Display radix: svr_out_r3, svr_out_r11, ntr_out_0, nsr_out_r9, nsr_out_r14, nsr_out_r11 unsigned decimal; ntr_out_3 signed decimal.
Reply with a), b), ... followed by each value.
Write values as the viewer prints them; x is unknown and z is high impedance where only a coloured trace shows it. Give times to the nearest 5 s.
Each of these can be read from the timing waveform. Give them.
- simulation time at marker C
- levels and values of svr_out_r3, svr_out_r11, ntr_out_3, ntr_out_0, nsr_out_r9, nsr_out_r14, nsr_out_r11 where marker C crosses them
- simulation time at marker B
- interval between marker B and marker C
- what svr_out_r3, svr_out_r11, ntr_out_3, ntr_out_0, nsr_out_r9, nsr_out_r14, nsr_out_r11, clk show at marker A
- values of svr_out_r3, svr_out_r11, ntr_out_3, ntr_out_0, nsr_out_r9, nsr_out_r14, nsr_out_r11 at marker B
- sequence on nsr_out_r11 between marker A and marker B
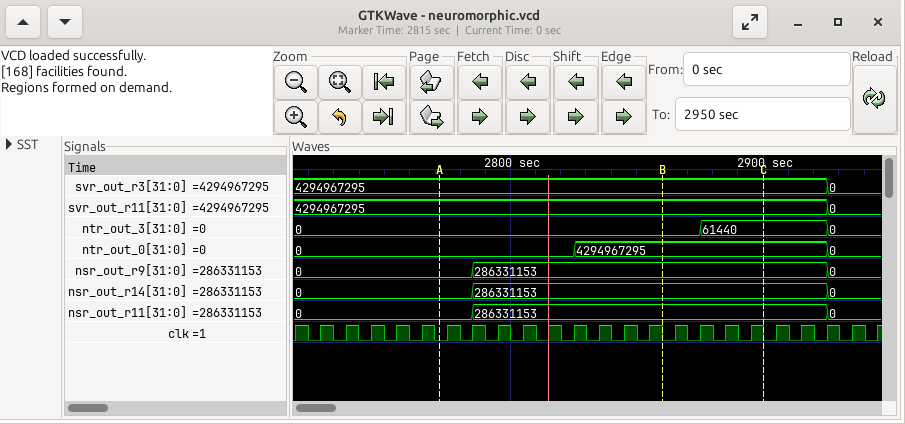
a) 2900 s
b) svr_out_r3=4294967295, svr_out_r11=4294967295, ntr_out_3=61440, ntr_out_0=4294967295, nsr_out_r9=286331153, nsr_out_r14=286331153, nsr_out_r11=286331153
c) 2860 s
d) 40 s
e) svr_out_r3=4294967295, svr_out_r11=4294967295, ntr_out_3=0, ntr_out_0=0, nsr_out_r9=0, nsr_out_r14=0, nsr_out_r11=0, clk=0
f) svr_out_r3=4294967295, svr_out_r11=4294967295, ntr_out_3=0, ntr_out_0=4294967295, nsr_out_r9=286331153, nsr_out_r14=286331153, nsr_out_r11=286331153
g) 0, 286331153
